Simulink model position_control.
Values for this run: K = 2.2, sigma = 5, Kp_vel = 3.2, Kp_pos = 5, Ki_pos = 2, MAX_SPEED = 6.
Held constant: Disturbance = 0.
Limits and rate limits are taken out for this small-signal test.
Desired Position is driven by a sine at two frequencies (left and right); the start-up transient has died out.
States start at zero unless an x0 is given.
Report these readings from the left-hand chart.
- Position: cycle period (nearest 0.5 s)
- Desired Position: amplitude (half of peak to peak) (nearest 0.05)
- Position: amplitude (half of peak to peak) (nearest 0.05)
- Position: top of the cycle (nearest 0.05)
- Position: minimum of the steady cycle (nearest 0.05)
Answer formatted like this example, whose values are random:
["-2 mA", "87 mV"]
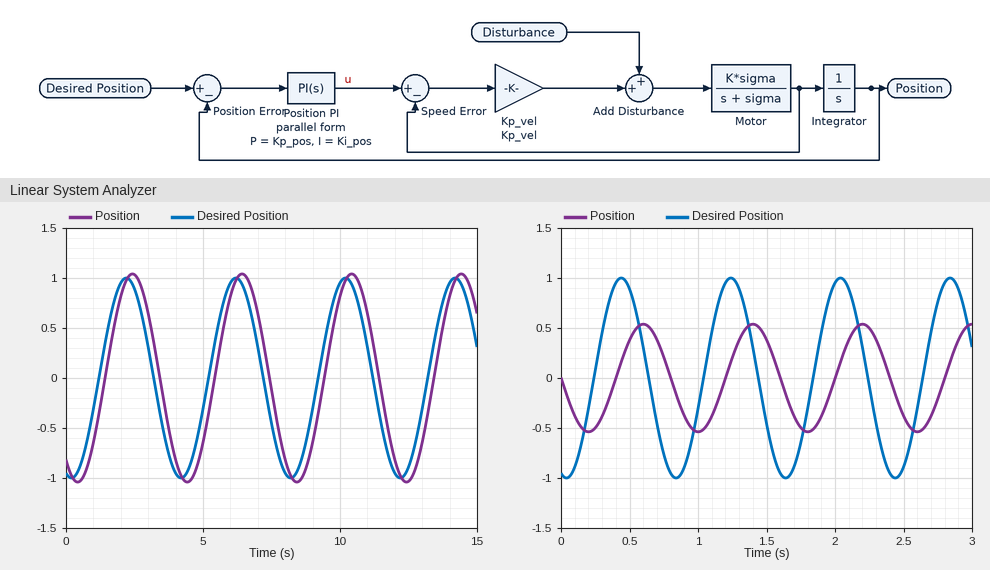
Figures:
["4.0 s", "1.00", "1.05", "1.05", "-1.05"]
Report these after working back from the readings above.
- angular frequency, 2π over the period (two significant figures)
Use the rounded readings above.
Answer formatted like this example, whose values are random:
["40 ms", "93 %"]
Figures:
["1.6 rad/s"]
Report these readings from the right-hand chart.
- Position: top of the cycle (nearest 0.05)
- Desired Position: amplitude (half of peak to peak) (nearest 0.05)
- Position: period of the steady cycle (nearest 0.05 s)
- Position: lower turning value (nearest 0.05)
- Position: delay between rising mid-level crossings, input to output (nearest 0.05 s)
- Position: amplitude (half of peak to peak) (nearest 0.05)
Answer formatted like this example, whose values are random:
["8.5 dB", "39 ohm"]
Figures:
["0.55", "1.00", "0.80 s", "-0.55", "0.15 s", "0.55"]
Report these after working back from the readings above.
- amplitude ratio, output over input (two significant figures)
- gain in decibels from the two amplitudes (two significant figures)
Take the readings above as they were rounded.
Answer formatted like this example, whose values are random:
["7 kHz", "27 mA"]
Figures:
["0.55", "-5.2 dB"]
